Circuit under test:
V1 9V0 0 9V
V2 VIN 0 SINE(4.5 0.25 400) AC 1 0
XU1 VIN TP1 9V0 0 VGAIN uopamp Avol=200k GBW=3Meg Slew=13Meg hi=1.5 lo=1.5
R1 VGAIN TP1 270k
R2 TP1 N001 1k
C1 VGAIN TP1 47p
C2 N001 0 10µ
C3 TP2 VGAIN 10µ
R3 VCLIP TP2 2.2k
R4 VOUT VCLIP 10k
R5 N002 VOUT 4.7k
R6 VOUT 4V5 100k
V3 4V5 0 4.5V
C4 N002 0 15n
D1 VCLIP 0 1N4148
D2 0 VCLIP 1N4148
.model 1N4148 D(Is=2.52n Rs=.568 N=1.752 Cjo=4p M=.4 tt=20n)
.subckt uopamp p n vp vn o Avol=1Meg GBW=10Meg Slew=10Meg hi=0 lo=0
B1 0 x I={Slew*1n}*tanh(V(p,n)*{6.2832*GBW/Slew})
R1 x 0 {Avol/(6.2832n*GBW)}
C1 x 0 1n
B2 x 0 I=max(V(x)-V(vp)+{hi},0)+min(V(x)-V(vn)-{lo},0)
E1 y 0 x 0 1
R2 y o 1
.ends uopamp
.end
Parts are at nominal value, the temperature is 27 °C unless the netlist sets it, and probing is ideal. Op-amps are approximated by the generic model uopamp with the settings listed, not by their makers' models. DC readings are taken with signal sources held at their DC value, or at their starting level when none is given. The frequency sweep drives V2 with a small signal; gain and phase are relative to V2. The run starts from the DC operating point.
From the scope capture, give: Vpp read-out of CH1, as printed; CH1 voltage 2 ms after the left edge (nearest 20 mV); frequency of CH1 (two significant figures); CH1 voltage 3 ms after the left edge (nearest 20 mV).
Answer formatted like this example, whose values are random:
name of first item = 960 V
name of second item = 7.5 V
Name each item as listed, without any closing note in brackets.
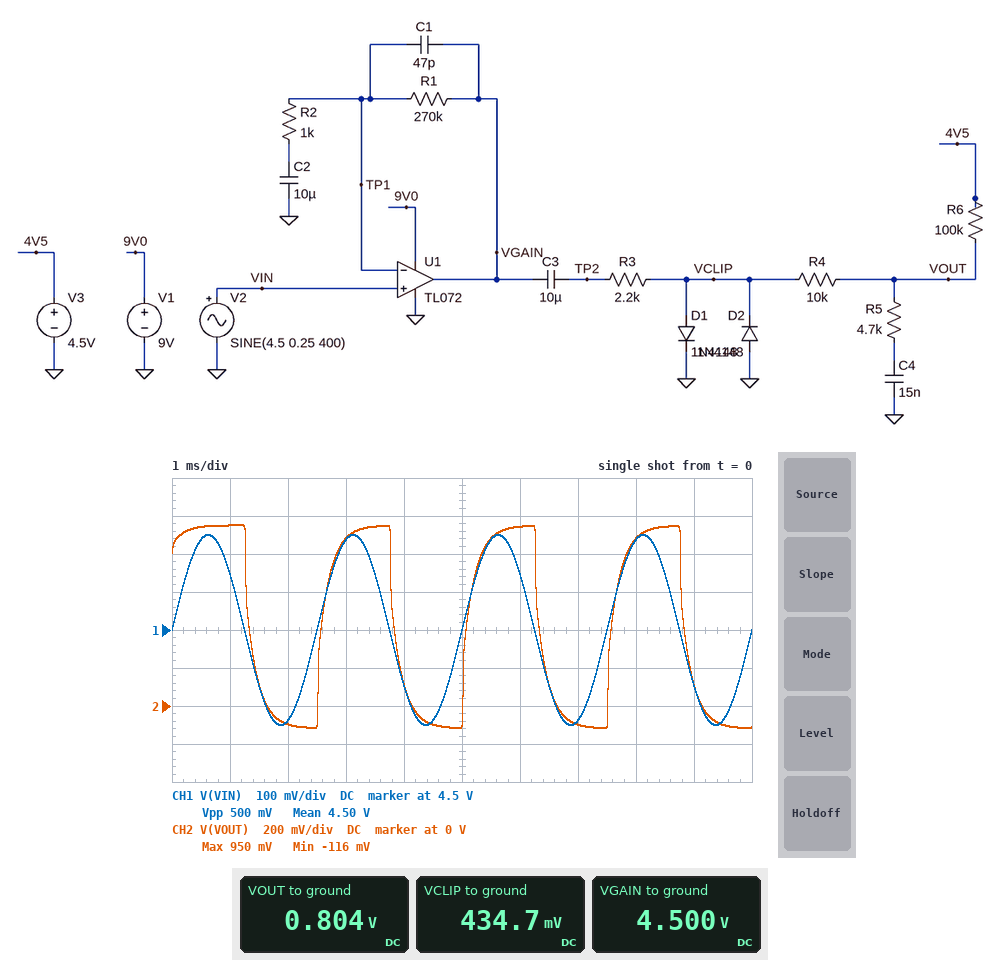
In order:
Vpp read-out of CH1, as printed = 500 mV
CH1 voltage 2 ms after the left edge = 4.26 V
frequency of CH1 = 400 Hz
CH1 voltage 3 ms after the left edge = 4.74 V
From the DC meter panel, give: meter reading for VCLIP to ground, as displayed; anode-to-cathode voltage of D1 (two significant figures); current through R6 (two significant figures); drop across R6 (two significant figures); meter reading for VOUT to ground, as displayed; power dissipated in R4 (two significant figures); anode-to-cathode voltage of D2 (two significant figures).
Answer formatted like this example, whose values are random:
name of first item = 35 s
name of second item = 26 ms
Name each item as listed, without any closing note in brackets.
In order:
meter reading for VCLIP to ground, as displayed = 434.7 mV
anode-to-cathode voltage of D1 = 430 mV
current through R6 = 37 µA
drop across R6 = 3.7 V
meter reading for VOUT to ground, as displayed = 0.804 V
power dissipated in R4 = 14 µW
anode-to-cathode voltage of D2 = -430 mV
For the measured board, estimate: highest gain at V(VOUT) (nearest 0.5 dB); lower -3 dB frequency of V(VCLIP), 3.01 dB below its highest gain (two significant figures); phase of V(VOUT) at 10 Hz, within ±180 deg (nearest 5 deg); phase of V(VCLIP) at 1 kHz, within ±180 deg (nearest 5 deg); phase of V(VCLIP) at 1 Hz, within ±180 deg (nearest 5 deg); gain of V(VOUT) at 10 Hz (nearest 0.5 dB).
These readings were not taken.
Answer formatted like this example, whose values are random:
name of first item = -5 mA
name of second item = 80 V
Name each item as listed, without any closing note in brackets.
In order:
highest gain at V(VOUT) = 38.5 dB
lower -3 dB frequency of V(VCLIP), 3.01 dB below its highest gain = 17 Hz
phase of V(VOUT) at 10 Hz, within ±180 deg = 80 deg
phase of V(VCLIP) at 1 kHz, within ±180 deg = -10 deg
phase of V(VCLIP) at 1 Hz, within ±180 deg = 160 deg
gain of V(VOUT) at 10 Hz = 32.5 dB
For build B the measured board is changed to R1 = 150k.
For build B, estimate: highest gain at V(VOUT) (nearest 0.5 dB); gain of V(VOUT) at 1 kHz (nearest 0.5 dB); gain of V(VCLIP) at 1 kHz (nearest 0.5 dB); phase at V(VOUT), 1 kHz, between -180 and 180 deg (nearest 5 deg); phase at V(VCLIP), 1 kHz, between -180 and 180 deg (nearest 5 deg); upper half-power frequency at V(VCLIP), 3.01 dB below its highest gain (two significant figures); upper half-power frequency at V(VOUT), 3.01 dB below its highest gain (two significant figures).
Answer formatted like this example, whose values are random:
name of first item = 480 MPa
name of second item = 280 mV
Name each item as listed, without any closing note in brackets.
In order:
highest gain at V(VOUT) = 33.5 dB
gain of V(VOUT) at 1 kHz = 30.0 dB
gain of V(VCLIP) at 1 kHz = 34.5 dB
phase at V(VOUT), 1 kHz, between -180 and 180 deg = -35 deg
phase at V(VCLIP), 1 kHz, between -180 and 180 deg = -5 deg
upper half-power frequency at V(VCLIP), 3.01 dB below its highest gain = 9.8 kHz
upper half-power frequency at V(VOUT), 3.01 dB below its highest gain = 860 Hz
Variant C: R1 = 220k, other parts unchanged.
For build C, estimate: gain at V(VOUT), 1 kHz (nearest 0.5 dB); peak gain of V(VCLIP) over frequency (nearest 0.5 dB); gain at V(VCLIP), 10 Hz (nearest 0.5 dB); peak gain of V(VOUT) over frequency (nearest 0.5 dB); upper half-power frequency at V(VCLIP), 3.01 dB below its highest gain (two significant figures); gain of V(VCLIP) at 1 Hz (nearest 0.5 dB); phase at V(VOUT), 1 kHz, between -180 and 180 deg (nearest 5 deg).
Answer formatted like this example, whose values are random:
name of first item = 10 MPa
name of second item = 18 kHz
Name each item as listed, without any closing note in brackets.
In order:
gain at V(VOUT), 1 kHz = 33.0 dB
peak gain of V(VCLIP) over frequency = 38.0 dB
gain at V(VCLIP), 10 Hz = 31.5 dB
peak gain of V(VOUT) over frequency = 37.0 dB
upper half-power frequency at V(VCLIP), 3.01 dB below its highest gain = 6.7 kHz
gain of V(VCLIP) at 1 Hz = 0.5 dB
phase at V(VOUT), 1 kHz, between -180 and 180 deg = -35 deg
